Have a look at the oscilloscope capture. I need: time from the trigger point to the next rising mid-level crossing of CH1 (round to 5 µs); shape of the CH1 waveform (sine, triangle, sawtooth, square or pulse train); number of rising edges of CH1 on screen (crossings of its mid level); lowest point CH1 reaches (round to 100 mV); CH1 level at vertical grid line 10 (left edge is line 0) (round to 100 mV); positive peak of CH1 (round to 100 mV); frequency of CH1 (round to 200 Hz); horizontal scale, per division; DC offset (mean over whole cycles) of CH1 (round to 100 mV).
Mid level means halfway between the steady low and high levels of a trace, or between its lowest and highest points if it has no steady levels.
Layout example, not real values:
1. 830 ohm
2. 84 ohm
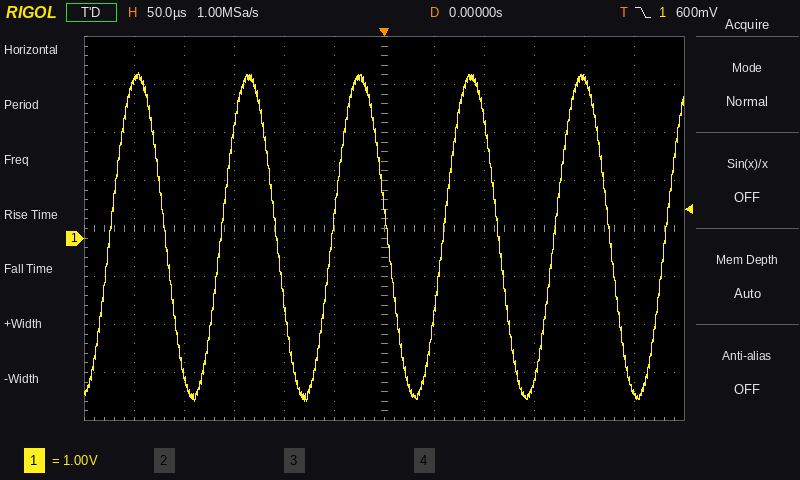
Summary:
1. 60 µs
2. sine
3. 6
4. -3.4 V
5. 3.3 V
6. 3.4 V
7. 9.0 kHz
8. 50 µs
9. 0.0 V
